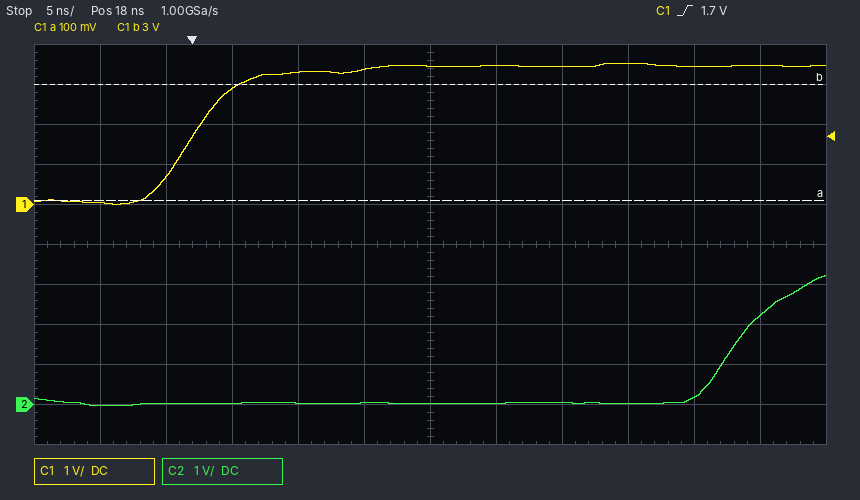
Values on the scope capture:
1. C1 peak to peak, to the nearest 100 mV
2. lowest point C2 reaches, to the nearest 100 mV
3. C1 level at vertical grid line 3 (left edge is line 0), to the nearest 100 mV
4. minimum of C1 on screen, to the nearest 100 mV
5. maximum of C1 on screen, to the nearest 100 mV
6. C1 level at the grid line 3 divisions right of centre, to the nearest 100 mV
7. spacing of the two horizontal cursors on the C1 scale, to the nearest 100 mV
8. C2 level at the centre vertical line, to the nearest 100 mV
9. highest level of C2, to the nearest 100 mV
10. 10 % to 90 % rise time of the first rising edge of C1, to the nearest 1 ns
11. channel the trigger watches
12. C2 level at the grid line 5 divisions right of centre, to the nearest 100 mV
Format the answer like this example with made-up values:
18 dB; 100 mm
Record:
3.5 V; 0.0 V; 2.9 V; 0.0 V; 3.5 V; 3.5 V; 2.9 V; 0.0 V; 3.2 V; 7 ns; C1; 2.2 V
